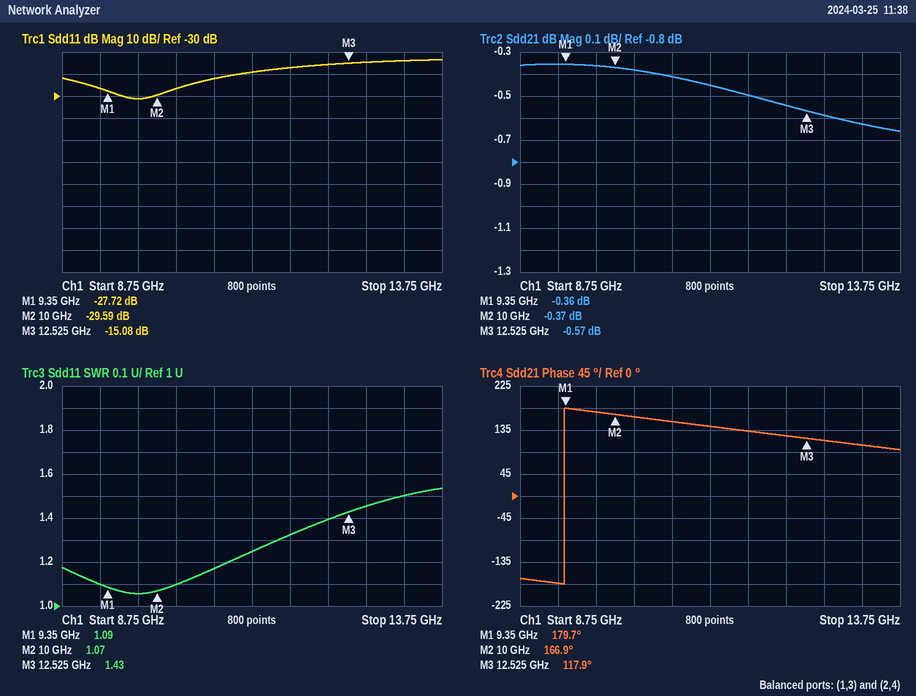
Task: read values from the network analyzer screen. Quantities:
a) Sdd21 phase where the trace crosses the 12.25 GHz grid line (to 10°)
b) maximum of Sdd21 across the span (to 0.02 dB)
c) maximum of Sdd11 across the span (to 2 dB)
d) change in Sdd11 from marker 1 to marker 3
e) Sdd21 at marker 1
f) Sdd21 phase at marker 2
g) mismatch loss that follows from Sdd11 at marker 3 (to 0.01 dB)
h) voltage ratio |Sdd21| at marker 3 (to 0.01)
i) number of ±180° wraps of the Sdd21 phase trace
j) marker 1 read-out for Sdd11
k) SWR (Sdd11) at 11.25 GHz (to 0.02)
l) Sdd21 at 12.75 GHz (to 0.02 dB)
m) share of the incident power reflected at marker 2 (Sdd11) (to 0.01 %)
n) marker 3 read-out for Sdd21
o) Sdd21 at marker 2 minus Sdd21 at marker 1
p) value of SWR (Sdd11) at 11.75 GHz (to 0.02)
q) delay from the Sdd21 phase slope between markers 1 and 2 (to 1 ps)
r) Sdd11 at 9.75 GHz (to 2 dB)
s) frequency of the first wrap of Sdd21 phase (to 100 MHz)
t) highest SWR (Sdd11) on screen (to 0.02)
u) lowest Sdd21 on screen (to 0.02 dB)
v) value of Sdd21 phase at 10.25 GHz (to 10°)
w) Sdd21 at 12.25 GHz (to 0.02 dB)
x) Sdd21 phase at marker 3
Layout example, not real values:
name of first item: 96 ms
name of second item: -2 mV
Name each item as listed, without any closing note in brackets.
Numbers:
Sdd21 phase where the trace crosses the 12.25 GHz grid line: 120°
maximum of Sdd21 across the span: -0.36 dB
maximum of Sdd11 across the span: -14 dB
change in Sdd11 from marker 1 to marker 3: 12.64 dB
Sdd21 at marker 1: -0.36 dB
Sdd21 phase at marker 2: 166.9°
mismatch loss that follows from Sdd11 at marker 3: 0.14 dB
voltage ratio |Sdd21| at marker 3: 0.94
number of ±180° wraps of the Sdd21 phase trace: 1
marker 1 read-out for Sdd11: -27.72 dB
SWR (Sdd11) at 11.25 GHz: 1.24
Sdd21 at 12.75 GHz: -0.58 dB
share of the incident power reflected at marker 2 (Sdd11): 0.11 %
marker 3 read-out for Sdd21: -0.57 dB
Sdd21 at marker 2 minus Sdd21 at marker 1: -0.01 dB
value of SWR (Sdd11) at 11.75 GHz: 1.32
delay from the Sdd21 phase slope between markers 1 and 2: 55 ps
Sdd11 at 9.75 GHz: -32 dB
frequency of the first wrap of Sdd21 phase: 9.3 GHz
highest SWR (Sdd11) on screen: 1.54
lowest Sdd21 on screen: -0.66 dB
value of Sdd21 phase at 10.25 GHz: 160°
Sdd21 at 12.25 GHz: -0.54 dB
Sdd21 phase at marker 3: 117.9°
